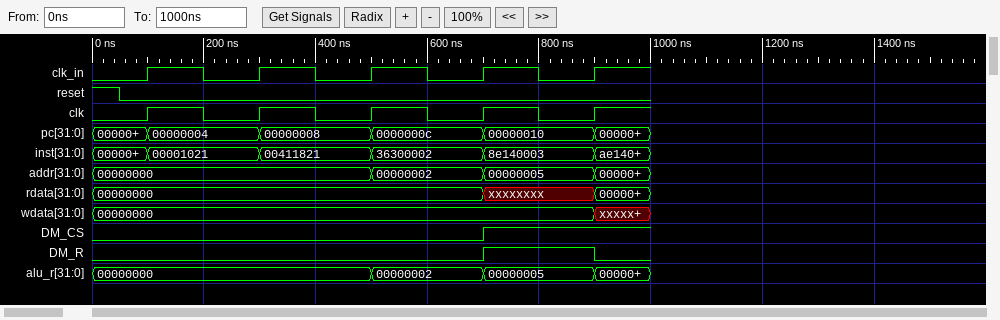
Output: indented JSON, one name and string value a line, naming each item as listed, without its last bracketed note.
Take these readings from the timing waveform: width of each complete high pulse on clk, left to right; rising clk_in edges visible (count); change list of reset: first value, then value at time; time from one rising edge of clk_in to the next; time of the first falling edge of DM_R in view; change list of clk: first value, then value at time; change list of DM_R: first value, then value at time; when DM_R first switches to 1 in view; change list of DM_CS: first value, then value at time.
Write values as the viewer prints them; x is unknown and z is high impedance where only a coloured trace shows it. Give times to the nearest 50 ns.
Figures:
{
  "width of each complete high pulse on clk, left to right": "100 ns, 100 ns, 100 ns, 100 ns",
  "rising clk_in edges visible": "5",
  "change list of reset: first value, then value at time": "1, 0 at 50 ns",
  "time from one rising edge of clk_in to the next": "200 ns",
  "time of the first falling edge of DM_R in view": "900 ns",
  "change list of clk: first value, then value at time": "0, 1 at 100 ns, 0 at 200 ns, 1 at 300 ns, 0 at 400 ns, 1 at 500 ns, 0 at 600 ns, 1 at 700 ns, 0 at 800 ns, 1 at 900 ns",
  "change list of DM_R: first value, then value at time": "0, 1 at 700 ns, 0 at 900 ns",
  "when DM_R first switches to 1 in view": "700 ns",
  "change list of DM_CS: first value, then value at time": "0, 1 at 700 ns"
}
